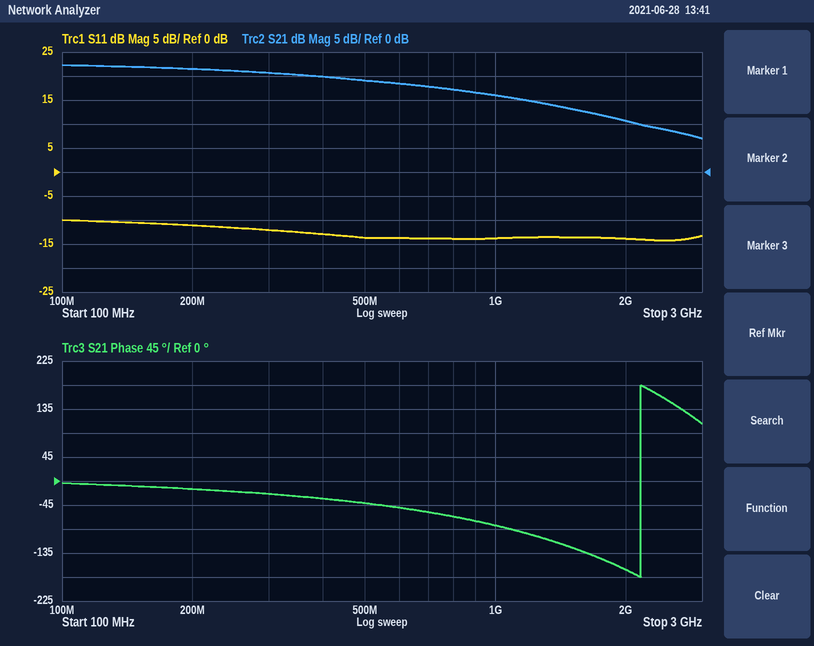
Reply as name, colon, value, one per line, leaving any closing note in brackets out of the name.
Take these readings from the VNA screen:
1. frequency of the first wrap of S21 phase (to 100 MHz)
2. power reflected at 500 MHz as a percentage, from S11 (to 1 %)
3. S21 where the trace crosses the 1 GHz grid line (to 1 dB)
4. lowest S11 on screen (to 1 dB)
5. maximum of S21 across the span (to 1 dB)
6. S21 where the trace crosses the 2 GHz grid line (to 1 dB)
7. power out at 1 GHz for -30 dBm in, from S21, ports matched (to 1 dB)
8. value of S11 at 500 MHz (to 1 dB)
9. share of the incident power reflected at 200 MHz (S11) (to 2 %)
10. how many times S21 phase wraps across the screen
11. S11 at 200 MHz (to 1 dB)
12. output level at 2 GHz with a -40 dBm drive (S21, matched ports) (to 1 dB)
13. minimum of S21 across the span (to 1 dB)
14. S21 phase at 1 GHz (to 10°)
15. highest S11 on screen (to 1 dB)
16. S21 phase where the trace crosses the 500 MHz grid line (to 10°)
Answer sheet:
frequency of the first wrap of S21 phase: 2.2 GHz
power reflected at 500 MHz as a percentage, from S11: 4 %
S21 where the trace crosses the 1 GHz grid line: 16 dB
lowest S11 on screen: -14 dB
maximum of S21 across the span: 22 dB
S21 where the trace crosses the 2 GHz grid line: 11 dB
power out at 1 GHz for -30 dBm in, from S21, ports matched: -14 dBm
value of S11 at 500 MHz: -14 dB
share of the incident power reflected at 200 MHz (S11): 8 %
how many times S21 phase wraps across the screen: 1
S11 at 200 MHz: -11 dB
output level at 2 GHz with a -40 dBm drive (S21, matched ports): -29 dBm
minimum of S21 across the span: 7 dB
S21 phase at 1 GHz: -80°
highest S11 on screen: -10 dB
S21 phase where the trace crosses the 500 MHz grid line: -40°
